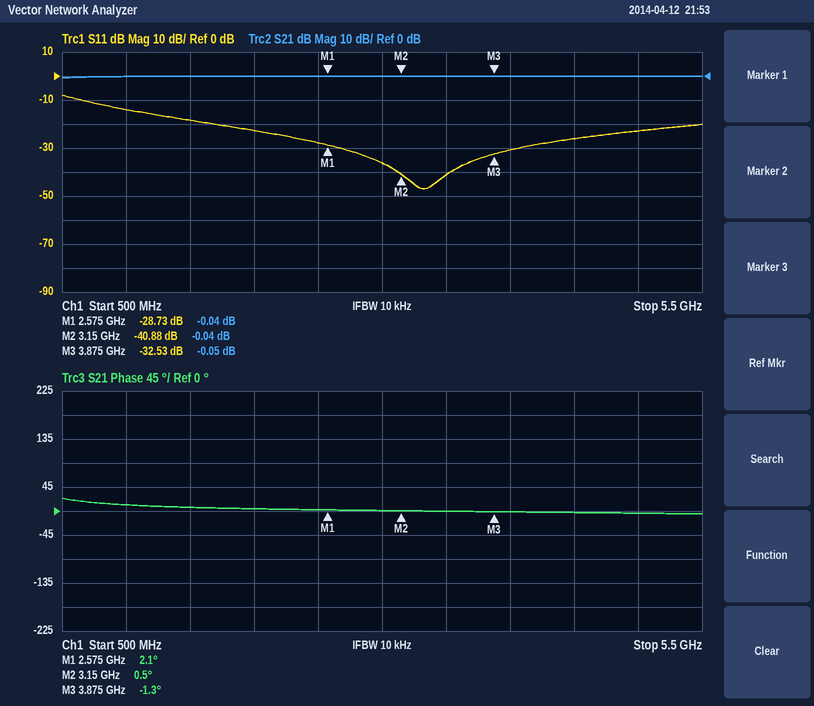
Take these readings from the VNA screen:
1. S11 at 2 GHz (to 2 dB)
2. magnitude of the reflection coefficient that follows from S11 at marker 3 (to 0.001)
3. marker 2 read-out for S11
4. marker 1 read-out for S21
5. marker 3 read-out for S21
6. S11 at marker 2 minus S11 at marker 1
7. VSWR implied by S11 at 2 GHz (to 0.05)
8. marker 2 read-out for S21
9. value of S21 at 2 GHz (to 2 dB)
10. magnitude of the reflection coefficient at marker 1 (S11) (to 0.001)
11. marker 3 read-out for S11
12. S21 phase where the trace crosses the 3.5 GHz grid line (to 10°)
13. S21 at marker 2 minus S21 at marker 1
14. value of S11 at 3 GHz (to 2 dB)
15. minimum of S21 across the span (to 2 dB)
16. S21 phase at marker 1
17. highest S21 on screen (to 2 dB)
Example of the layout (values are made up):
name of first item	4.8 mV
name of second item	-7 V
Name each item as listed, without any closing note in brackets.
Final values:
S11 at 2 GHz	-22 dB
magnitude of the reflection coefficient that follows from S11 at marker 3	0.024
marker 2 read-out for S11	-40.88 dB
marker 1 read-out for S21	-0.04 dB
marker 3 read-out for S21	-0.05 dB
S11 at marker 2 minus S11 at marker 1	-12.15 dB
VSWR implied by S11 at 2 GHz	1.15
marker 2 read-out for S21	-0.04 dB
value of S21 at 2 GHz	0 dB
magnitude of the reflection coefficient at marker 1 (S11)	0.037
marker 3 read-out for S11	-32.53 dB
S21 phase where the trace crosses the 3.5 GHz grid line	0°
S21 at marker 2 minus S21 at marker 1	0.00 dB
value of S11 at 3 GHz	-36 dB
minimum of S21 across the span	0 dB
S21 phase at marker 1	2.1°
highest S21 on screen	0 dB
